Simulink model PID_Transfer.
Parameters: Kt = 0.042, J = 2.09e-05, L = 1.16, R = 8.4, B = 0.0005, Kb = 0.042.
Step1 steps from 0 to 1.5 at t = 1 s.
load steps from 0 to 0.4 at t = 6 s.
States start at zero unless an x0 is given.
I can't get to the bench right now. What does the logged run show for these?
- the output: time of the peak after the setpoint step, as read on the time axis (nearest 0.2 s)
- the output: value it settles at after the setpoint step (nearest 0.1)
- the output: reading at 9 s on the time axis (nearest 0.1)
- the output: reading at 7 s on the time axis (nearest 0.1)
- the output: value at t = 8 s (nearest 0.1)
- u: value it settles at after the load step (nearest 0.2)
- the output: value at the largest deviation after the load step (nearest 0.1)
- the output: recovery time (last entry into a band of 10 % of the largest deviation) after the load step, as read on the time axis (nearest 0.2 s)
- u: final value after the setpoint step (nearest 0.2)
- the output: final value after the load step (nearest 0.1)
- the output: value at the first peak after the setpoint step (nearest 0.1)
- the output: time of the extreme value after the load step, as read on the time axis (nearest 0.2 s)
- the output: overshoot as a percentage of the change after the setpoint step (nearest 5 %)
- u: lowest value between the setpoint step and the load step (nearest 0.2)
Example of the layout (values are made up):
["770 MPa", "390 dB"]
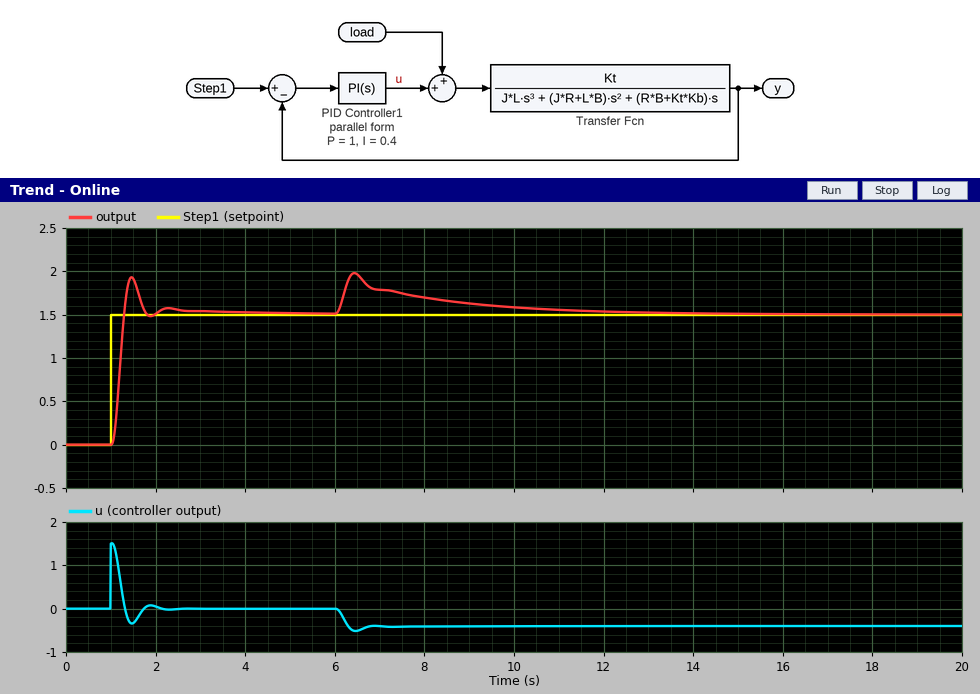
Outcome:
["1.4 s", "1.5", "1.6", "1.8", "1.7", "-0.4", "2.0", "11.4 s", "0.0", "1.5", "1.9", "6.4 s", "30 %", "-0.4"]
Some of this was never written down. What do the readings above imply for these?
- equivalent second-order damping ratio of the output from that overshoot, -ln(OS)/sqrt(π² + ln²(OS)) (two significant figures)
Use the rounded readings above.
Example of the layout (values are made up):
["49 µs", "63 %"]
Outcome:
["0.36"]
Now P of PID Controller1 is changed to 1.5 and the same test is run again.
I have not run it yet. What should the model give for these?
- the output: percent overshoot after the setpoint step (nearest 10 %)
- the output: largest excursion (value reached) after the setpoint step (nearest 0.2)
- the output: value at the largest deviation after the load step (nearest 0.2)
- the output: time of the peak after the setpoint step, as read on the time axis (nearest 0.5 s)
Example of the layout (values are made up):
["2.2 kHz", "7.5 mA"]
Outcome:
["40 %", "2.2", "1.8", "1.5 s"]
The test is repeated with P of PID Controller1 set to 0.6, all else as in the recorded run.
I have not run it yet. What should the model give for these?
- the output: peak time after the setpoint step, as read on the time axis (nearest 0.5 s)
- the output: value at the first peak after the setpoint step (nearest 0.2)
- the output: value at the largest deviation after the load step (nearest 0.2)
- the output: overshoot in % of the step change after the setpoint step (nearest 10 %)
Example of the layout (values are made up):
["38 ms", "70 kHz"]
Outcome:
["1.5 s", "1.8", "2.2", "20 %"]
